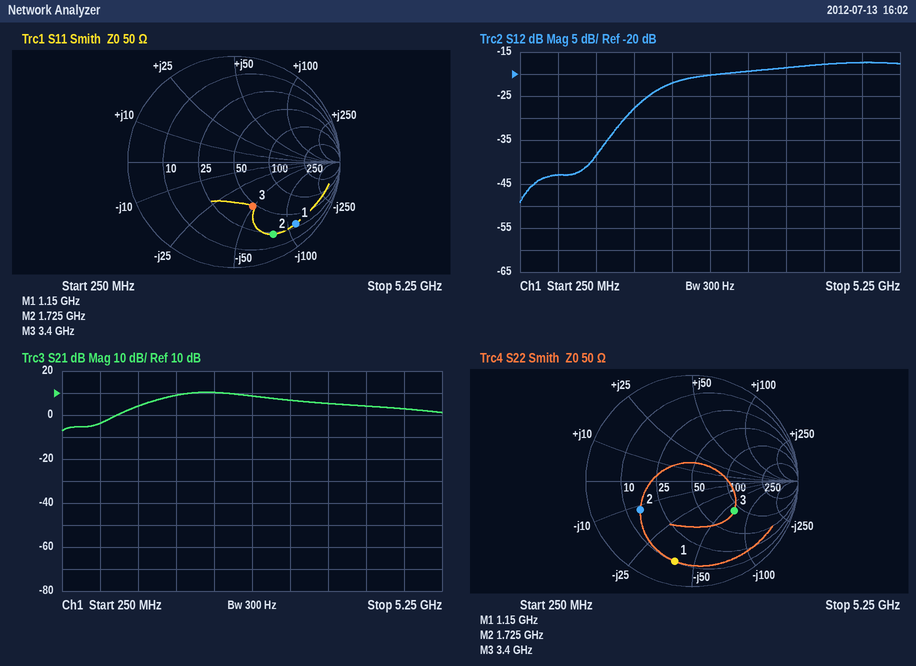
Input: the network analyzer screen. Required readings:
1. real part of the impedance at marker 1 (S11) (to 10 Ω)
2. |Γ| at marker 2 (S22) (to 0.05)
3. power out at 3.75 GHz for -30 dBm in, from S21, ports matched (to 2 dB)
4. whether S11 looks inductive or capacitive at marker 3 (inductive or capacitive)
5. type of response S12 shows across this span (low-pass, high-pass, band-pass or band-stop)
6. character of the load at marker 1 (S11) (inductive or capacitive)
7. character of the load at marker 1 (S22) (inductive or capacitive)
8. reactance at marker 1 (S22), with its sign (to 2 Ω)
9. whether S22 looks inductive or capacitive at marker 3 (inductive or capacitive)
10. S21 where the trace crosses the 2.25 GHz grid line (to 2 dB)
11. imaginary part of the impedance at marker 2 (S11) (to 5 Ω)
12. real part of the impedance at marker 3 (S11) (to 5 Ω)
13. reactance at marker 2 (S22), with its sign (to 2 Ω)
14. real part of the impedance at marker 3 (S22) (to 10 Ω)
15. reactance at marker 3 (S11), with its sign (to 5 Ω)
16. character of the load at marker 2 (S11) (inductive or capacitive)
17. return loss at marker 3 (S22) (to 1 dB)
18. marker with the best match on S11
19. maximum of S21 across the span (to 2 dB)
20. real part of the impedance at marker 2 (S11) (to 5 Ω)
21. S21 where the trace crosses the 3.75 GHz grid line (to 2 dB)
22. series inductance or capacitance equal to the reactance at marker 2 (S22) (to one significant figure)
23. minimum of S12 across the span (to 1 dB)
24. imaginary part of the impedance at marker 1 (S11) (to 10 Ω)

30 Ω
0.55
-24 dBm
capacitive
high-pass
capacitive
capacitive
-40 Ω
capacitive
10 dB
-80 Ω
45 Ω
-12 Ω
90 Ω
-50 Ω
capacitive
6 dB
marker 3
10 dB
25 Ω
6 dB
8 pF
-49 dB
-110 Ω
